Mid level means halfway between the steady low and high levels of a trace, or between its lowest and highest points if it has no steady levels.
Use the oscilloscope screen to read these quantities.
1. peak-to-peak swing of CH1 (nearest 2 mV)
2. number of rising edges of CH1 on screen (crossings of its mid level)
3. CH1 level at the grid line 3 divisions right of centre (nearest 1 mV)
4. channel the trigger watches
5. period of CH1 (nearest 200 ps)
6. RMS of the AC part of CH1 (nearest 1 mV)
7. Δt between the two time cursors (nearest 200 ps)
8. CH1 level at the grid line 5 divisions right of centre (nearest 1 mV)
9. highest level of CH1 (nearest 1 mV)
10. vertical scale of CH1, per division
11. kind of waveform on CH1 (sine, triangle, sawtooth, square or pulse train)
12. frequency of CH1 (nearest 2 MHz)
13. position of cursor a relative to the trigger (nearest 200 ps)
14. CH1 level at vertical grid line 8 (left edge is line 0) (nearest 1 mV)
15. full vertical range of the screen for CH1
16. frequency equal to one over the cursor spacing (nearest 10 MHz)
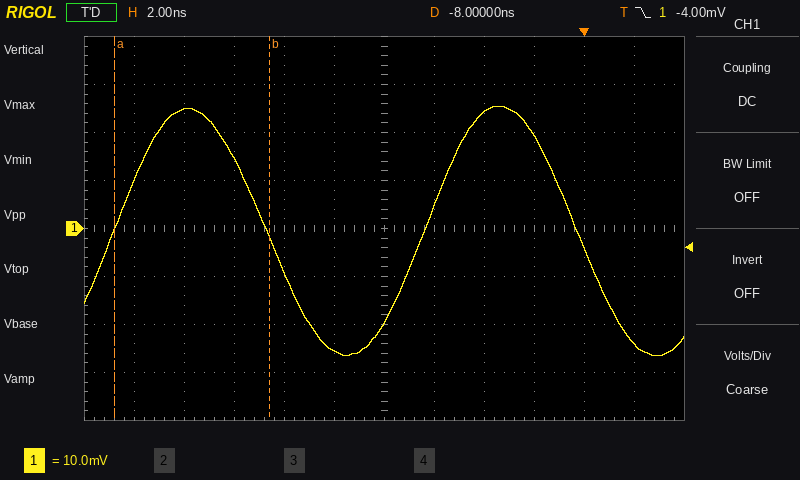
52 mV
2
19 mV
CH1
12.4 ns
18 mV
6.2 ns
-24 mV
25 mV
10 mV
sine
80 MHz
-18.8 ns
24 mV
80 mV
160 MHz
